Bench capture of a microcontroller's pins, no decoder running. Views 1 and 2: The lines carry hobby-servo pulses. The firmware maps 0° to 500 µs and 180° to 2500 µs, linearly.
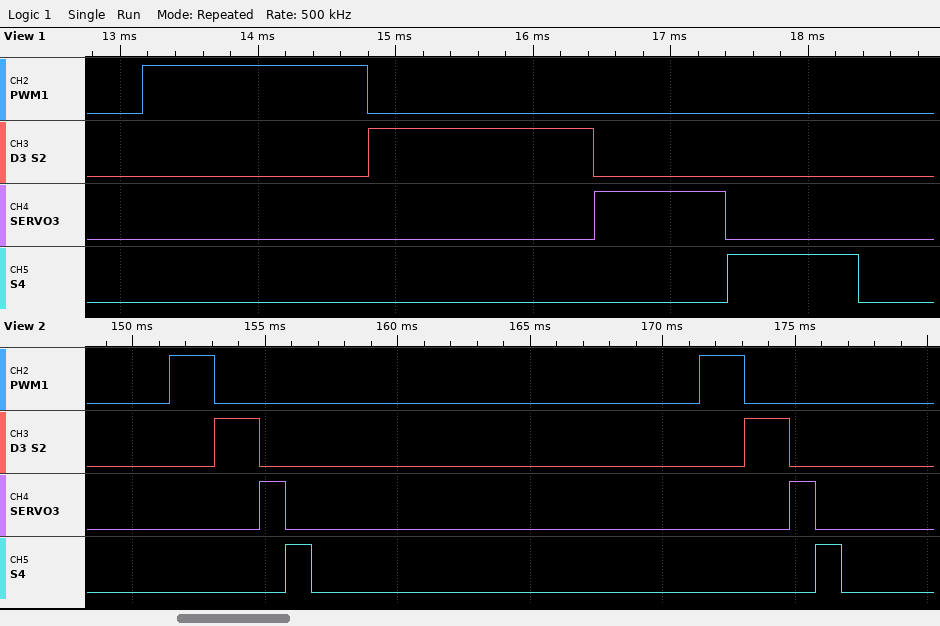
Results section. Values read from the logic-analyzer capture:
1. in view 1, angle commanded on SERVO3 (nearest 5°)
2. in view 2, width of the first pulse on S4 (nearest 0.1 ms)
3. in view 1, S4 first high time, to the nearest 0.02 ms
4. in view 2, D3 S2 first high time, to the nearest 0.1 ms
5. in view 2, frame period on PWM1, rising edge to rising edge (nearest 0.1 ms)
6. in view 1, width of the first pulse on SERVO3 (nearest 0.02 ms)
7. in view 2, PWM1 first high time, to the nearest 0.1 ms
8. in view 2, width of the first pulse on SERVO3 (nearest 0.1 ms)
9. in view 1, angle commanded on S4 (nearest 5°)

40°
1.0 ms
0.96 ms
1.7 ms
20.0 ms
0.96 ms
1.7 ms
1.0 ms
40°
